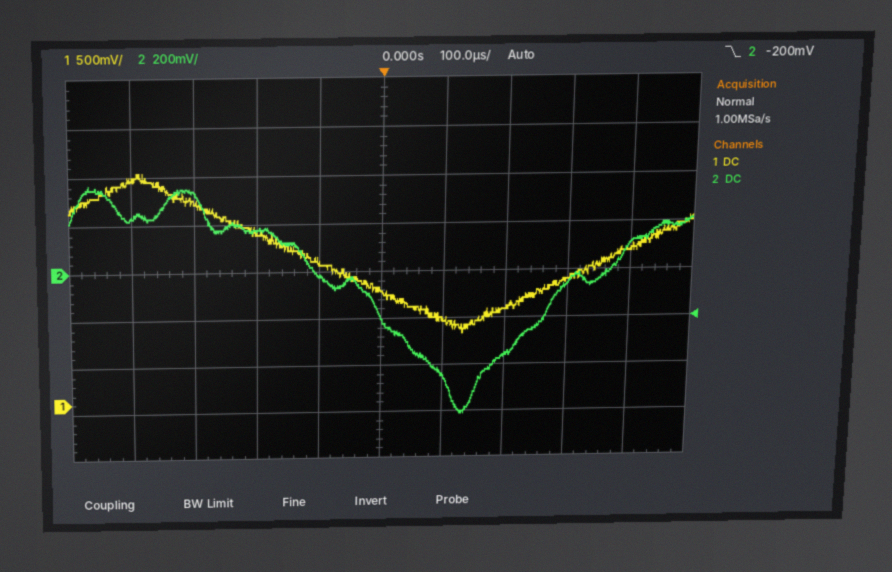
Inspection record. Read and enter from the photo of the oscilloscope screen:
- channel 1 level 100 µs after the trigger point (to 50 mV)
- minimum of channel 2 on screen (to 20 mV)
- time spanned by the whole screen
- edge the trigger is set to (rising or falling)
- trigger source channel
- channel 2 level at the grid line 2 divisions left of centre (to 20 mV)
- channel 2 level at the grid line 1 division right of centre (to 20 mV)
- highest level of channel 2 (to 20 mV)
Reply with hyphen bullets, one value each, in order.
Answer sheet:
- 900 mV
- -600 mV
- 1 ms
- falling
- channel 2
- 180 mV
- -440 mV
- 360 mV
